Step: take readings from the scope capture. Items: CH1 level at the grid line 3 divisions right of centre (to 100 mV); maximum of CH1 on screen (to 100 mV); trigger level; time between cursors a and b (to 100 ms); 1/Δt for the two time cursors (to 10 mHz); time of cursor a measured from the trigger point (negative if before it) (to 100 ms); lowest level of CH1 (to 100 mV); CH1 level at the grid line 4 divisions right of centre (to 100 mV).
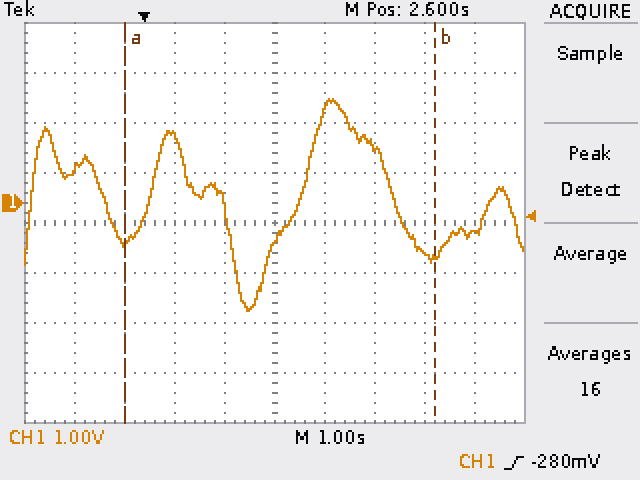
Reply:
-1.0 V
2.1 V
-280 mV
6.2 s
160 mHz
-400 ms
-2.2 V
-600 mV
